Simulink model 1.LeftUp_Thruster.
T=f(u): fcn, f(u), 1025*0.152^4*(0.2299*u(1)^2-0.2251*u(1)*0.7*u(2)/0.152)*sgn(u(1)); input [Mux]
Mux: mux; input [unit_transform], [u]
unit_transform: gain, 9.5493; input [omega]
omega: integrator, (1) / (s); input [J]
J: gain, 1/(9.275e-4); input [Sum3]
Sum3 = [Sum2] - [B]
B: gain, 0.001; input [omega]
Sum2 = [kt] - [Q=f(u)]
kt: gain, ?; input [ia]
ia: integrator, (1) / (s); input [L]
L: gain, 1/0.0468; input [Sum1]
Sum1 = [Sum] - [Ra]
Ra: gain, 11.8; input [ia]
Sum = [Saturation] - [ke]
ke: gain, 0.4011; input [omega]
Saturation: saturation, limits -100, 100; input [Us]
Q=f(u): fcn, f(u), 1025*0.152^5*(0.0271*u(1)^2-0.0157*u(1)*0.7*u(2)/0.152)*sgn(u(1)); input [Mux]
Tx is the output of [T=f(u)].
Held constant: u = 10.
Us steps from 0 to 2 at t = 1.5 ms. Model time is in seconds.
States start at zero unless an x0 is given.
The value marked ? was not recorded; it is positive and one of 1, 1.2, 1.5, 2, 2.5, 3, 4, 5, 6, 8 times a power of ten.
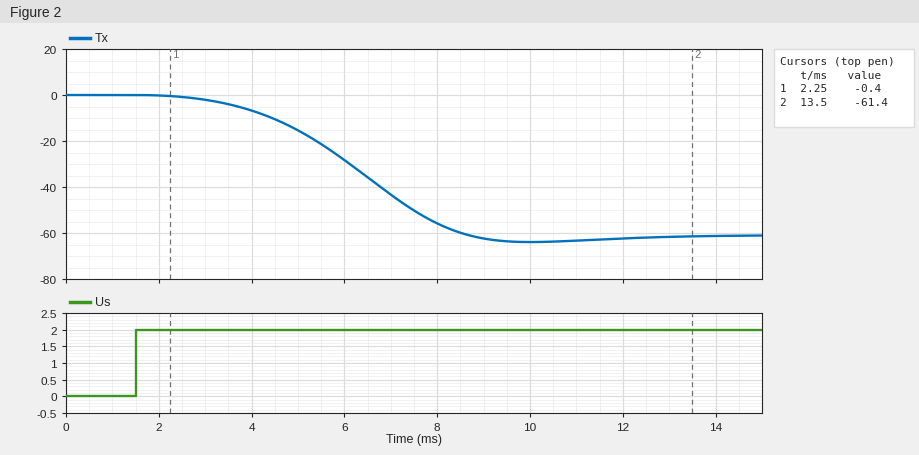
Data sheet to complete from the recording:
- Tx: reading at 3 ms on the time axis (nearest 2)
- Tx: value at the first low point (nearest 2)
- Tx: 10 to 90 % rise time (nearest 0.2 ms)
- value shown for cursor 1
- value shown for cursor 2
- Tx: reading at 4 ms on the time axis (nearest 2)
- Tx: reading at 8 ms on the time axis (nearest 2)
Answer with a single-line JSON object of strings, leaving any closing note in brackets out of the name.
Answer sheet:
{"Tx: reading at 3 ms on the time axis": "-2", "Tx: value at the first low point": "-64", "Tx: 10 to 90 % rise time": "4.0 ms", "value shown for cursor 1": "-0.4", "value shown for cursor 2": "-61.4", "Tx: reading at 4 ms on the time axis": "-6", "Tx: reading at 8 ms on the time axis": "-56"}
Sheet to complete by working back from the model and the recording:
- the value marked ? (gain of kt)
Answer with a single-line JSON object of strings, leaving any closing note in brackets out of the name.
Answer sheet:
{"the value marked ?": "0.6"}
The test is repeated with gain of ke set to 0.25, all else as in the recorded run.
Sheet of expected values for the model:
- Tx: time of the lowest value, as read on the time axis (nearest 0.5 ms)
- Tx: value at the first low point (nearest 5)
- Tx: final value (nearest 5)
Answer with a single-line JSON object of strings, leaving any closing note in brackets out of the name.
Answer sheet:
{"Tx: time of the lowest value, as read on the time axis": "10.0 ms", "Tx: value at the first low point": "-65", "Tx: final value": "-60"}
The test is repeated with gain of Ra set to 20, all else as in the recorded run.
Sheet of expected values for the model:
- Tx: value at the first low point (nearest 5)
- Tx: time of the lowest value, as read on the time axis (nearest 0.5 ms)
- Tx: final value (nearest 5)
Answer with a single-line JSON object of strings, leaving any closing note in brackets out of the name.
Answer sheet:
{"Tx: value at the first low point": "-65", "Tx: time of the lowest value, as read on the time axis": "10.5 ms", "Tx: final value": "-60"}
